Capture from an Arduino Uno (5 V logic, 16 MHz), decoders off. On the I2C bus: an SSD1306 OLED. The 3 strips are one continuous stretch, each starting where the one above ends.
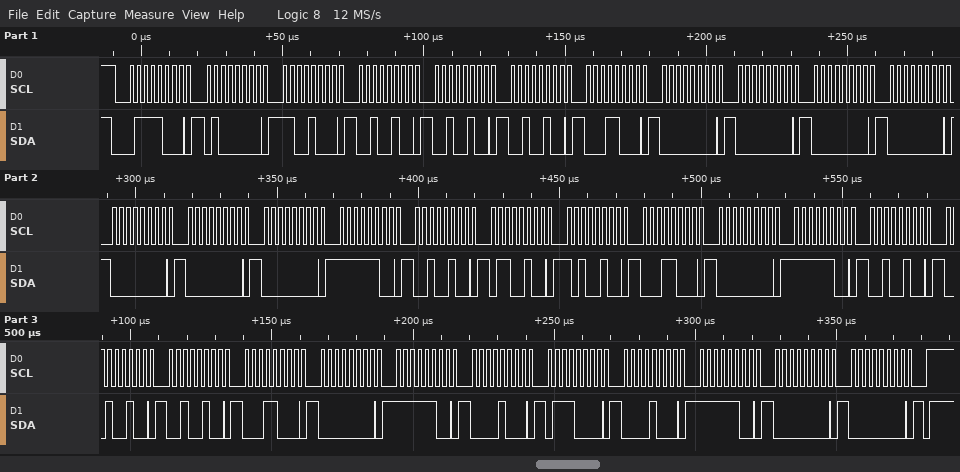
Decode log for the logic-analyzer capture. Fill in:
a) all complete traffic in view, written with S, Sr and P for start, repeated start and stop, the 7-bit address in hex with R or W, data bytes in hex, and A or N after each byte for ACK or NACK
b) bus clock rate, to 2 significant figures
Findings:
S 3CW A 40 A C8 A 24 A 24 A 24 A 18 A 00 A 00 A 00 A 00 A 00 A 00 A 00 A FC A 24 A 64 A A4 A 18 A 00 A FC A 24 A 24 A 24 A 18 A 00 A FC A 08 A 70 A 08 A FC A 00 A 00 A P
400 kHz
